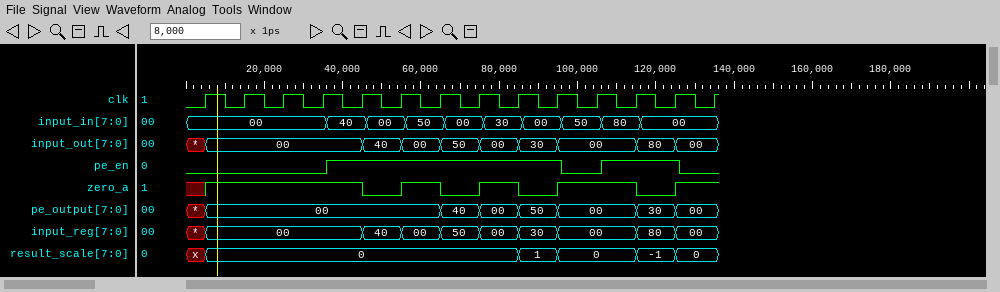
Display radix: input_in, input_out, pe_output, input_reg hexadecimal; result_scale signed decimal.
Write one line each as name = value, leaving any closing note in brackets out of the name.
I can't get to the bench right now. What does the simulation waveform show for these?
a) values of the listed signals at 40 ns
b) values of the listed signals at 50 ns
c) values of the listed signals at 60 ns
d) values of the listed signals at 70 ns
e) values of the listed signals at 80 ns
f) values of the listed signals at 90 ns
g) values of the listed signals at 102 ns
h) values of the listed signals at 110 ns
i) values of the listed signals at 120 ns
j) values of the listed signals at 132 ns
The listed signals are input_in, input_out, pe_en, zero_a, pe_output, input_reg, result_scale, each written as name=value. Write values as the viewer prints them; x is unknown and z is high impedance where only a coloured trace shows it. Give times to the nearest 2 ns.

values of the listed signals at 40 ns = input_in=40, input_out=00, pe_en=1, zero_a=1, pe_output=00, input_reg=00, result_scale=0
values of the listed signals at 50 ns = input_in=00, input_out=40, pe_en=1, zero_a=0, pe_output=00, input_reg=40, result_scale=0
values of the listed signals at 60 ns = input_in=50, input_out=00, pe_en=1, zero_a=1, pe_output=00, input_reg=00, result_scale=0
values of the listed signals at 70 ns = input_in=00, input_out=50, pe_en=1, zero_a=0, pe_output=40, input_reg=50, result_scale=0
values of the listed signals at 80 ns = input_in=30, input_out=00, pe_en=1, zero_a=1, pe_output=00, input_reg=00, result_scale=0
values of the listed signals at 90 ns = input_in=00, input_out=30, pe_en=1, zero_a=0, pe_output=50, input_reg=30, result_scale=1
values of the listed signals at 102 ns = input_in=50, input_out=00, pe_en=0, zero_a=1, pe_output=00, input_reg=00, result_scale=0
values of the listed signals at 110 ns = input_in=80, input_out=00, pe_en=1, zero_a=1, pe_output=00, input_reg=00, result_scale=0
values of the listed signals at 120 ns = input_in=00, input_out=80, pe_en=1, zero_a=0, pe_output=30, input_reg=80, result_scale=-1
values of the listed signals at 132 ns = input_in=00, input_out=00, pe_en=0, zero_a=1, pe_output=00, input_reg=00, result_scale=0
